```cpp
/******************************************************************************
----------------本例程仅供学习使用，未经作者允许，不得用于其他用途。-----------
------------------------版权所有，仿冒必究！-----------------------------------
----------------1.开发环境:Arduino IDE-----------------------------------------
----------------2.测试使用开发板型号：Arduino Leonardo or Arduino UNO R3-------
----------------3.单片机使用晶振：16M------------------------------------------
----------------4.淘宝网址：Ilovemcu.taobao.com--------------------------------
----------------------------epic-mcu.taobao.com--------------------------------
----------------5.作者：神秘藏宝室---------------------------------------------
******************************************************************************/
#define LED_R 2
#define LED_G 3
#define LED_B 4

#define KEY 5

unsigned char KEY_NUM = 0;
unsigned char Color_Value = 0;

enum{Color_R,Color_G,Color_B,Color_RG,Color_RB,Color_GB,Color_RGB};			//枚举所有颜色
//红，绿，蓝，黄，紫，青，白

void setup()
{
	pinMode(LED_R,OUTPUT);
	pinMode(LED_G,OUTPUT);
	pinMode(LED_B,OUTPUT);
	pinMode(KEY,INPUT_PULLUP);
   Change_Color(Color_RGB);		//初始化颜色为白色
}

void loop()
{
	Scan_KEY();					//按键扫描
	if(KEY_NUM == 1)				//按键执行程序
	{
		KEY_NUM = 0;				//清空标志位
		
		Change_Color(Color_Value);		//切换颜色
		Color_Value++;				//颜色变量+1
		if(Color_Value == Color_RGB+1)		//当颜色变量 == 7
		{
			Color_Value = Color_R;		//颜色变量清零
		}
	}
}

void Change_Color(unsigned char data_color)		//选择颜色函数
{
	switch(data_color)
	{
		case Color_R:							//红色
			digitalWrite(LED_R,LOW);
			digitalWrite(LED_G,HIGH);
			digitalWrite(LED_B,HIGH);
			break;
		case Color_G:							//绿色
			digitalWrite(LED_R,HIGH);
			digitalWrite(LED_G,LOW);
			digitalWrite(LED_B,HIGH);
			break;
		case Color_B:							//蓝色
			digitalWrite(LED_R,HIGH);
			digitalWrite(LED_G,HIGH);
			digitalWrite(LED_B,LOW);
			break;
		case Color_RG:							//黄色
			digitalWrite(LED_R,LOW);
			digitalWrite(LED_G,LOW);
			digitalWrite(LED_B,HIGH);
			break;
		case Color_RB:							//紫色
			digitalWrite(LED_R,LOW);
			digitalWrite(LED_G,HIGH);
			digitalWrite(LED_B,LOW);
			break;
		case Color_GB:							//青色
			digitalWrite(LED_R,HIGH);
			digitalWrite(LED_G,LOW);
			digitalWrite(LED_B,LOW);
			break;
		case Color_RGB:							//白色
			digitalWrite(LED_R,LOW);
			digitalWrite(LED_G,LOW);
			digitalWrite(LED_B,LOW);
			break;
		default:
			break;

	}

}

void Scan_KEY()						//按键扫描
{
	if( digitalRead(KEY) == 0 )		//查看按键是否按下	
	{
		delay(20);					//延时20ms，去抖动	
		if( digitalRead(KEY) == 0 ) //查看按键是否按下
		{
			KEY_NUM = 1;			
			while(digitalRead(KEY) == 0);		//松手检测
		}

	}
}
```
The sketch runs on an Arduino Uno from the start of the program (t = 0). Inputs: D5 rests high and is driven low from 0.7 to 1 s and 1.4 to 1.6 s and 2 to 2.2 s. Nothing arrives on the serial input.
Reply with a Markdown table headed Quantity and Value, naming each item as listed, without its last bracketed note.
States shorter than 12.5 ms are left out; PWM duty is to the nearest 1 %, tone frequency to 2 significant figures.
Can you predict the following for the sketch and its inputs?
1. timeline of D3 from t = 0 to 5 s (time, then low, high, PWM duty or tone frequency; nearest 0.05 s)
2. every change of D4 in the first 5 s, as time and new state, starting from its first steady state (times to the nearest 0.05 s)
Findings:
| Quantity | Value |
|---|---|
| timeline of D3 from t = 0 to 5 s | 0 s low; 1 s high; 1.6 s low; 2.2 s high |
| every change of D4 in the first 5 s, as time and new state, starting from its first steady state | 0 s low; 1 s high; 2.2 s low |
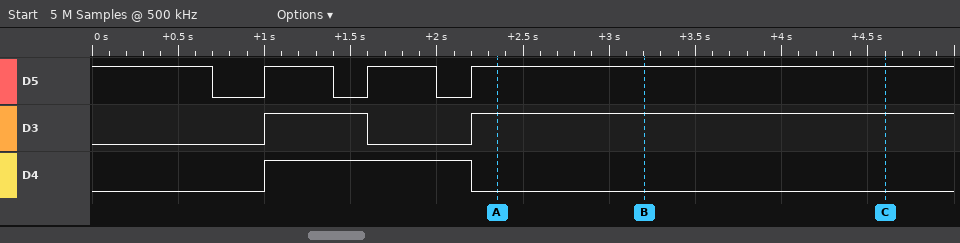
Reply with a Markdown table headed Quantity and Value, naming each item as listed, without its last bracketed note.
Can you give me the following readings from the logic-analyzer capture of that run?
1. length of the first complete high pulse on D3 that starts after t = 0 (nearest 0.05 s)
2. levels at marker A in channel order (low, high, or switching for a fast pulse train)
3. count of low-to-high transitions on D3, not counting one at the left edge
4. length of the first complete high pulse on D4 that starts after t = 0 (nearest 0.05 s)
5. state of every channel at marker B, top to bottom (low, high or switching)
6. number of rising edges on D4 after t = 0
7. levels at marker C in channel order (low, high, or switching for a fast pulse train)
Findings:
| Quantity | Value |
|---|---|
| length of the first complete high pulse on D3 that starts after t = 0 | 0.60 s |
| levels at marker A in channel order | D5 high, D3 high, D4 low |
| count of low-to-high transitions on D3, not counting one at the left edge | 2 |
| length of the first complete high pulse on D4 that starts after t = 0 | 1.20 s |
| state of every channel at marker B, top to bottom | D5 high, D3 high, D4 low |
| number of rising edges on D4 after t = 0 | 1 |
| levels at marker C in channel order | D5 high, D3 high, D4 low |
